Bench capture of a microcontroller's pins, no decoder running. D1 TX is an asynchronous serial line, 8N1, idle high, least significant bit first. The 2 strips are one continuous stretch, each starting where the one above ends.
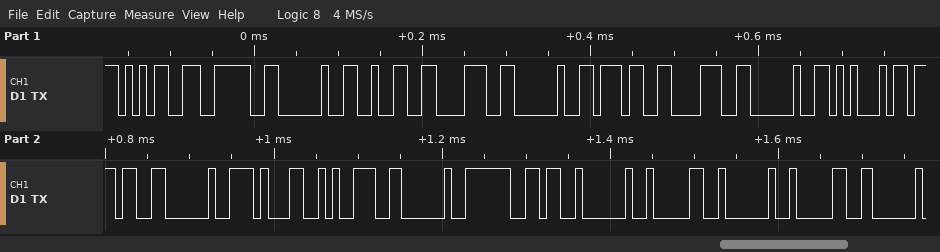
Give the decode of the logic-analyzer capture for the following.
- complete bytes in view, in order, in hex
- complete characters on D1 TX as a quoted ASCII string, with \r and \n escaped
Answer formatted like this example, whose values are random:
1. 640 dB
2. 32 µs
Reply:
1. 0x35 0x3E 0x20 0x32 0x38 0x20 0x37 0x38 0x20 0x45 0x37 0x20 0x31 0x39 0x20 0x36 0x20 0x30 0x20 0x30
2. "5> 28 78 E7 19 6 0 0"
